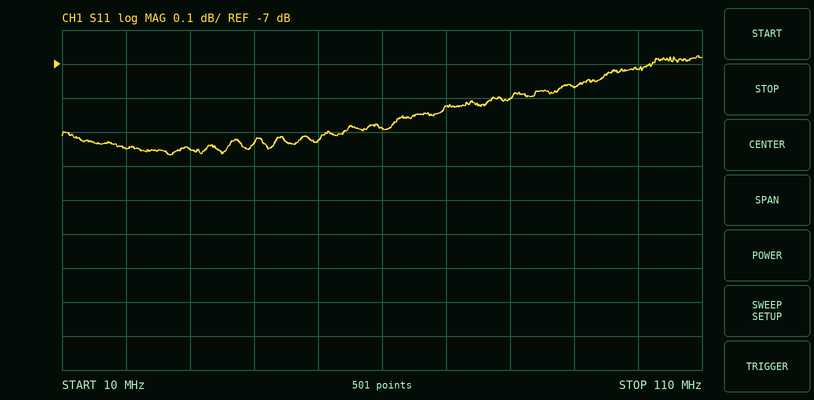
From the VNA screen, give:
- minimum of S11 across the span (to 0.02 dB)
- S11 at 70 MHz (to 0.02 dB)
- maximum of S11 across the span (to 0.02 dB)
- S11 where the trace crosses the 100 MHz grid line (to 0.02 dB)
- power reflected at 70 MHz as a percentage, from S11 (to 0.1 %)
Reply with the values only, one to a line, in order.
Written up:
-7.26 dB
-7.12 dB
-6.98 dB
-7.02 dB
19.4 %
